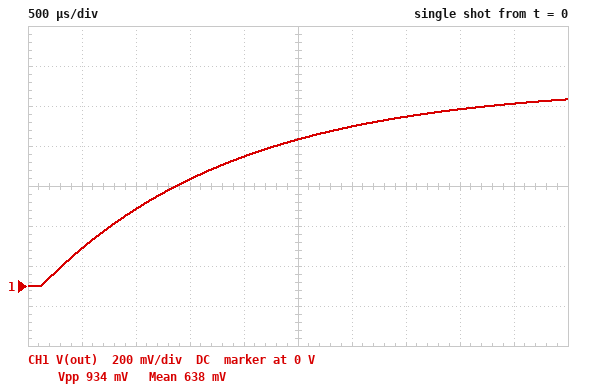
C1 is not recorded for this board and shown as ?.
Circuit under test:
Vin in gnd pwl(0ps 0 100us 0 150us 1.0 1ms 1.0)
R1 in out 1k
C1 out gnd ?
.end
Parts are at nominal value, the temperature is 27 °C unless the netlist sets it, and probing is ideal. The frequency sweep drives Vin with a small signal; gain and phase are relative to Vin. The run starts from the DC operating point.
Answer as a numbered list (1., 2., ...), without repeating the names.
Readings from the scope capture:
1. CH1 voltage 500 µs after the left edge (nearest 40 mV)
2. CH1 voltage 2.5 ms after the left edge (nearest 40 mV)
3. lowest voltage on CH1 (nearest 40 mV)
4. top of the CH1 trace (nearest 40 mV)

1. 200 mV
2. 720 mV
3. 0 V
4. 920 mV
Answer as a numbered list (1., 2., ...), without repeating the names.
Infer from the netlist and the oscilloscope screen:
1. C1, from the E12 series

1. 1.8 µF
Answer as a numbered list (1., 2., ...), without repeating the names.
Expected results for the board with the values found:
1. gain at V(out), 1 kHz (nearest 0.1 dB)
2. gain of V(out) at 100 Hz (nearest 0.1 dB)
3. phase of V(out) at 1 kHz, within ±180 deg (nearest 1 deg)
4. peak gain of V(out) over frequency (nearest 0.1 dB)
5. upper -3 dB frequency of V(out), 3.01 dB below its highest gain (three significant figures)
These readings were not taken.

1. -21.1 dB
2. -3.6 dB
3. -85 deg
4. 0 dB
5. 88.4 Hz
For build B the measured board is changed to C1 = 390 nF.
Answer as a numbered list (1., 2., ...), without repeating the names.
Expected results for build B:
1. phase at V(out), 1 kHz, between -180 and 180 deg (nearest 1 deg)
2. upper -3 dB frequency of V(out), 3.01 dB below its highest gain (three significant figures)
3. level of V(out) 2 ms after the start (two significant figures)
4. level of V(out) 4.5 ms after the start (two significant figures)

1. -68 deg
2. 408 Hz
3. 990 mV
4. 1.0 V
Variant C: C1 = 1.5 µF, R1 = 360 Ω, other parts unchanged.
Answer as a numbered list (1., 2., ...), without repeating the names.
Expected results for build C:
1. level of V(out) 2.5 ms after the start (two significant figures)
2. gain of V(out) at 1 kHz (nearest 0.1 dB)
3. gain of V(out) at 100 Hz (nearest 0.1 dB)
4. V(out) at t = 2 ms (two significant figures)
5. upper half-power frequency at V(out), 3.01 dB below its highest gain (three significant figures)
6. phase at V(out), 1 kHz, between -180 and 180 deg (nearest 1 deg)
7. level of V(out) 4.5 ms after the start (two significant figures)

1. 990 mV
2. -11.0 dB
3. -0.5 dB
4. 970 mV
5. 295 Hz
6. -74 deg
7. 1.0 V
